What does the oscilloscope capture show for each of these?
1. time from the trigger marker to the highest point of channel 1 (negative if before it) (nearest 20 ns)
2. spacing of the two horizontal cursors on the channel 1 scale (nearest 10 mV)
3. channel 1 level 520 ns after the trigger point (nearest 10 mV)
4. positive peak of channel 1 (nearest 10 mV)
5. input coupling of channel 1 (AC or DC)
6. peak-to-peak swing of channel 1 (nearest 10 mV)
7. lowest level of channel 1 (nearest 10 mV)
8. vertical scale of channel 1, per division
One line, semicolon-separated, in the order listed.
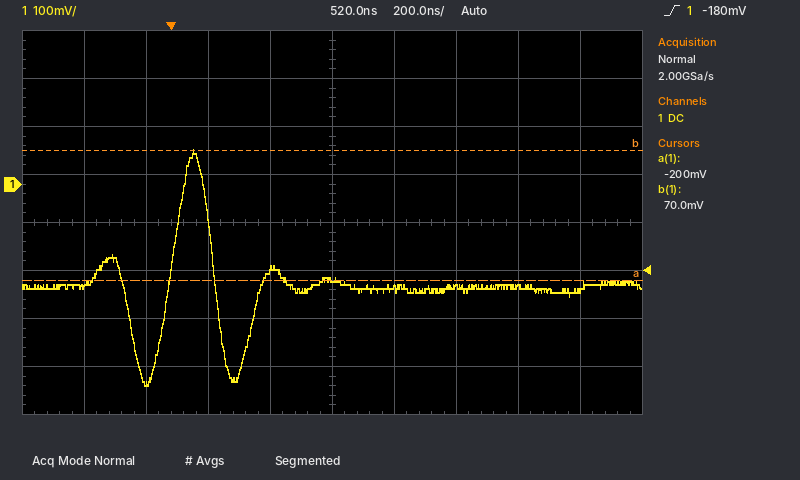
+80 ns; 270 mV; -200 mV; 70 mV; DC; 490 mV; -420 mV; 100 mV
